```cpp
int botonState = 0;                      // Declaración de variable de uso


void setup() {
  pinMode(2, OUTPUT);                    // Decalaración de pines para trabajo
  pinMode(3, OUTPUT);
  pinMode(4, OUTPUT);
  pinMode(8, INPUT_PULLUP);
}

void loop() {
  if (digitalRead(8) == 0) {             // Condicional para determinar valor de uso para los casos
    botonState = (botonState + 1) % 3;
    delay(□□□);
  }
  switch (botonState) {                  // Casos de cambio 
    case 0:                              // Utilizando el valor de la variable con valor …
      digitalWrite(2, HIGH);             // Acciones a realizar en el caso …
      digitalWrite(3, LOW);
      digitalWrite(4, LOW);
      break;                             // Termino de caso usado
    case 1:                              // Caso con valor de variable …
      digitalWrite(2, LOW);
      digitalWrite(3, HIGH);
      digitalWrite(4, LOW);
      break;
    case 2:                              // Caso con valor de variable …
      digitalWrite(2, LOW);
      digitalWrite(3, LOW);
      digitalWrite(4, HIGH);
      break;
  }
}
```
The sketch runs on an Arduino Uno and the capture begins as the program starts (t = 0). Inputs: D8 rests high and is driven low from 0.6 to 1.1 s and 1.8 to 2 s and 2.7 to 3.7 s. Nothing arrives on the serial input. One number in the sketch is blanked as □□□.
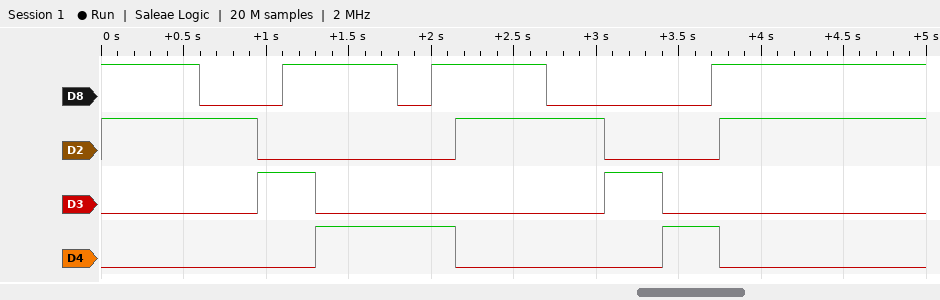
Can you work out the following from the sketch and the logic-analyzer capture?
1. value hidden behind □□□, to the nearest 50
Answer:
350
